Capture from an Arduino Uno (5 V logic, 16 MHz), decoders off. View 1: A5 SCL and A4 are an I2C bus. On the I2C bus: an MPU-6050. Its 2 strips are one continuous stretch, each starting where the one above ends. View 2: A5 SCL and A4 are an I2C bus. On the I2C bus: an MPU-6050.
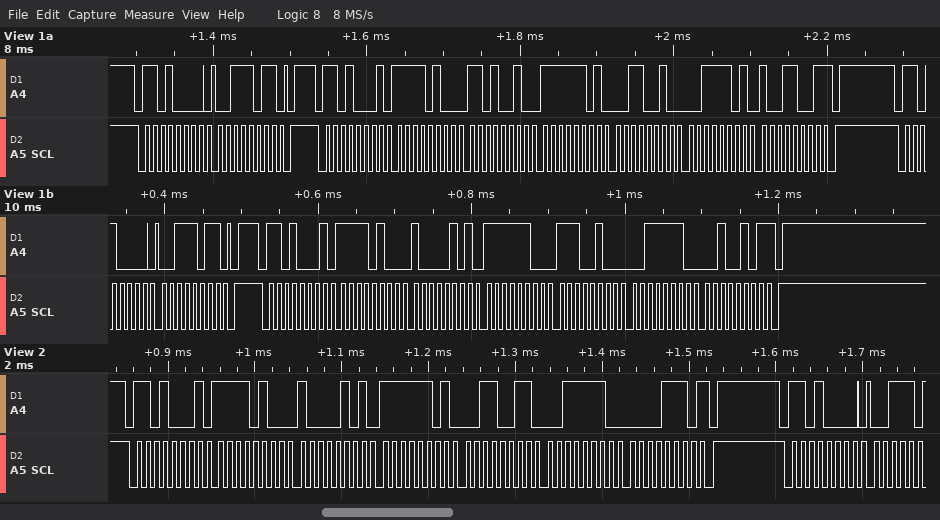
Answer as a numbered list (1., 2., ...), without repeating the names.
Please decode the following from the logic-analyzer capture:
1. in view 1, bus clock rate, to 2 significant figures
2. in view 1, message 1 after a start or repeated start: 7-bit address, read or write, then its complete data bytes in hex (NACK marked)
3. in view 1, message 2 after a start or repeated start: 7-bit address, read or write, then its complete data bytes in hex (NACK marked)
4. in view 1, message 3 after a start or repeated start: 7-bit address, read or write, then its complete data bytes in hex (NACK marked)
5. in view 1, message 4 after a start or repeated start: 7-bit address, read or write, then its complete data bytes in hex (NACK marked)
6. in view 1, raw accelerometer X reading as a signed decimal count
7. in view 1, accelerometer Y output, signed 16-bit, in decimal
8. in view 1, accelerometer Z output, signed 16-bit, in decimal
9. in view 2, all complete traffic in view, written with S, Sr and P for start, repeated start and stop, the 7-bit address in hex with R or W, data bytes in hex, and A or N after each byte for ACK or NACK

1. 100 kHz
2. 0x68 write: 3B
3. 0x68 read: F4 D2 FD 32 3D 99 NACK
4. 0x68 write: 3B
5. 0x68 read: F4 85 FC E4 3E 25 NACK
6. -2862
7. -718
8. 15769
9. S 68R A F4 A 85 A FD A 33 A 3E A 0E N P S 68W A
